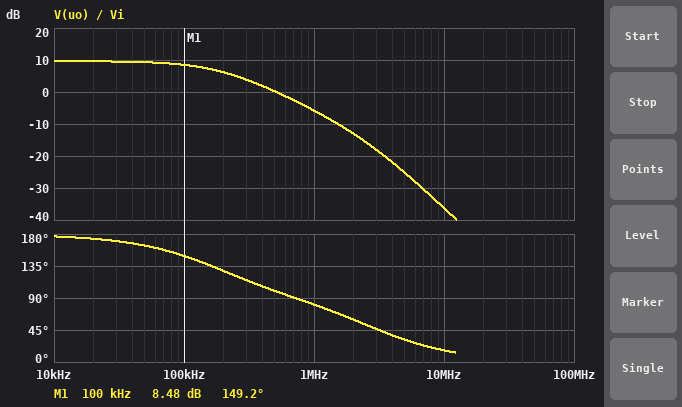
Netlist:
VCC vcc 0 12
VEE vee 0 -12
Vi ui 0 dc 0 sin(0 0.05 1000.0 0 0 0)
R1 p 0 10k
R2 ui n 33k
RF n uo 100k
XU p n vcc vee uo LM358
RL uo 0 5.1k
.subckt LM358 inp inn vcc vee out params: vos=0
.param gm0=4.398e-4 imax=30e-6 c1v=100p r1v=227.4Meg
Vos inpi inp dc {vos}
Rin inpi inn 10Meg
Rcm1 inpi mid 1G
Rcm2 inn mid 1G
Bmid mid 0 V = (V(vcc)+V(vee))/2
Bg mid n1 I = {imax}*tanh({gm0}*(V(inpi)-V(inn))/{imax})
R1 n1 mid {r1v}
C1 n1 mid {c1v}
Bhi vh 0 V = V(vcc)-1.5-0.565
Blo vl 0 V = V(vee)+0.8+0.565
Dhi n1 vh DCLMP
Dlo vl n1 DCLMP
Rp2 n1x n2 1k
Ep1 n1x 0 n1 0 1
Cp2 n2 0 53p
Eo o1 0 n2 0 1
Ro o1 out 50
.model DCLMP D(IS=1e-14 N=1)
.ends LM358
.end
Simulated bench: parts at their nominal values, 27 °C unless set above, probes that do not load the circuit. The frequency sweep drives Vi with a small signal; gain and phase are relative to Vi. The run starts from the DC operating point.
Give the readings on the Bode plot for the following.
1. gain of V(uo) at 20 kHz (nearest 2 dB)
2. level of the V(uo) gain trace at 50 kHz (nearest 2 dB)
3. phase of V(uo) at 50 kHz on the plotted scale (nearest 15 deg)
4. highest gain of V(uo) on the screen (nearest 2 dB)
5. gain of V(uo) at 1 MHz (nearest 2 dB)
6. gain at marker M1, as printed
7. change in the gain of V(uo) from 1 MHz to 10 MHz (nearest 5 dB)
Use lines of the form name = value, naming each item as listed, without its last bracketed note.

gain of V(uo) at 20 kHz = 10 dB
level of the V(uo) gain trace at 50 kHz = 10 dB
phase of V(uo) at 50 kHz on the plotted scale = 165 deg
highest gain of V(uo) on the screen = 10 dB
gain of V(uo) at 1 MHz = -6 dB
gain at marker M1, as printed = 8.48 dB
change in the gain of V(uo) from 1 MHz to 10 MHz = -30 dB
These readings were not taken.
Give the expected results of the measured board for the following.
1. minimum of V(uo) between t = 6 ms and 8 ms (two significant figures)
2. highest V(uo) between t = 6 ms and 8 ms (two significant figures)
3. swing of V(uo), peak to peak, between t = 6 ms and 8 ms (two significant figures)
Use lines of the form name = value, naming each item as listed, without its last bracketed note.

minimum of V(uo) between t = 6 ms and 8 ms = -150 mV
highest V(uo) between t = 6 ms and 8 ms = 150 mV
swing of V(uo), peak to peak, between t = 6 ms and 8 ms = 300 mV
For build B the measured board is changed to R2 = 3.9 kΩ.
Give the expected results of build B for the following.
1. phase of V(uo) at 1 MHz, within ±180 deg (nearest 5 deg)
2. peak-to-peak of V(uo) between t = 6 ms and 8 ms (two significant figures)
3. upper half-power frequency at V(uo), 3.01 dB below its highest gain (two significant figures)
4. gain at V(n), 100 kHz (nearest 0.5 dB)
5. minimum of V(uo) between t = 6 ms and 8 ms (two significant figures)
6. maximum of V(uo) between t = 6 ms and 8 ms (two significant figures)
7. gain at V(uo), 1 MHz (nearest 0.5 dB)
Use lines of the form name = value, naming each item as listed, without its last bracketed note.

phase of V(uo) at 1 MHz, within ±180 deg = 75 deg
peak-to-peak of V(uo) between t = 6 ms and 8 ms = 2.6 V
upper half-power frequency at V(uo), 3.01 dB below its highest gain = 26 kHz
gain at V(n), 100 kHz = -0.5 dB
minimum of V(uo) between t = 6 ms and 8 ms = -1.3 V
maximum of V(uo) between t = 6 ms and 8 ms = 1.3 V
gain at V(uo), 1 MHz = -4.0 dB
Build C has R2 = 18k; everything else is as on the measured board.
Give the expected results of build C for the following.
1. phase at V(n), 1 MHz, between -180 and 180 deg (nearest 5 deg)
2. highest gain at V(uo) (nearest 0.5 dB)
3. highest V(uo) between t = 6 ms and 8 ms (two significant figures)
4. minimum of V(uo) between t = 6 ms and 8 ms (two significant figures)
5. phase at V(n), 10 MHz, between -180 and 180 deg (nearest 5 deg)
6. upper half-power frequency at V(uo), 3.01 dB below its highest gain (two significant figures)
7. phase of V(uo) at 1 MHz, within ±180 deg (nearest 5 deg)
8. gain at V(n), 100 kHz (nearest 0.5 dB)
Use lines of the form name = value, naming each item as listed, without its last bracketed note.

phase at V(n), 1 MHz, between -180 and 180 deg = 5 deg
highest gain at V(uo) = 15.0 dB
highest V(uo) between t = 6 ms and 8 ms = 280 mV
minimum of V(uo) between t = 6 ms and 8 ms = -280 mV
phase at V(n), 10 MHz, between -180 and 180 deg = 0 deg
upper half-power frequency at V(uo), 3.01 dB below its highest gain = 110 kHz
phase of V(uo) at 1 MHz, within ±180 deg = 75 deg
gain at V(n), 100 kHz = -4.5 dB
